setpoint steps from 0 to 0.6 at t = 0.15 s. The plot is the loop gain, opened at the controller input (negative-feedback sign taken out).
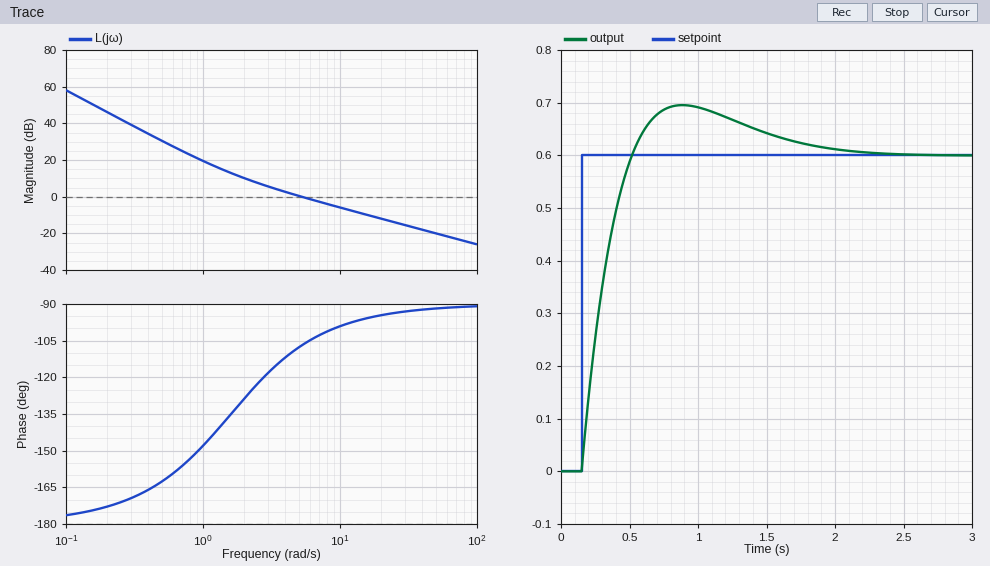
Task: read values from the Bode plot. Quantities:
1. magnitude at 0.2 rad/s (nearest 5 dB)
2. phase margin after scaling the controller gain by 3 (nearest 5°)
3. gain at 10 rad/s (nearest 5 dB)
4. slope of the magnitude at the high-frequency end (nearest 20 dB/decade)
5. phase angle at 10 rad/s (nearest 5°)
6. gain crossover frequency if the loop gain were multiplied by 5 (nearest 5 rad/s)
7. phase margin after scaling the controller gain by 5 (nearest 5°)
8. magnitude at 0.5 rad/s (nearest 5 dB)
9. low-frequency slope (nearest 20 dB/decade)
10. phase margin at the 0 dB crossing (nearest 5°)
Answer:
45 dB
85°
-5 dB
-20 dB/decade
-100°
25 rad/s
85°
30 dB
-40 dB/decade
75°
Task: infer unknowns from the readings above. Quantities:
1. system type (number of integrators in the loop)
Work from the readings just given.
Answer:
2
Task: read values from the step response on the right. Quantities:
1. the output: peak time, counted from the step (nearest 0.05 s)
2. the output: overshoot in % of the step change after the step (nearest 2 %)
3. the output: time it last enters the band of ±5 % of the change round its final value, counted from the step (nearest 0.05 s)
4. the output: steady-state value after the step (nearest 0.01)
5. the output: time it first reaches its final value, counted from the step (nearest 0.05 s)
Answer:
0.75 s
16 %
1.50 s
0.60
0.35 s
